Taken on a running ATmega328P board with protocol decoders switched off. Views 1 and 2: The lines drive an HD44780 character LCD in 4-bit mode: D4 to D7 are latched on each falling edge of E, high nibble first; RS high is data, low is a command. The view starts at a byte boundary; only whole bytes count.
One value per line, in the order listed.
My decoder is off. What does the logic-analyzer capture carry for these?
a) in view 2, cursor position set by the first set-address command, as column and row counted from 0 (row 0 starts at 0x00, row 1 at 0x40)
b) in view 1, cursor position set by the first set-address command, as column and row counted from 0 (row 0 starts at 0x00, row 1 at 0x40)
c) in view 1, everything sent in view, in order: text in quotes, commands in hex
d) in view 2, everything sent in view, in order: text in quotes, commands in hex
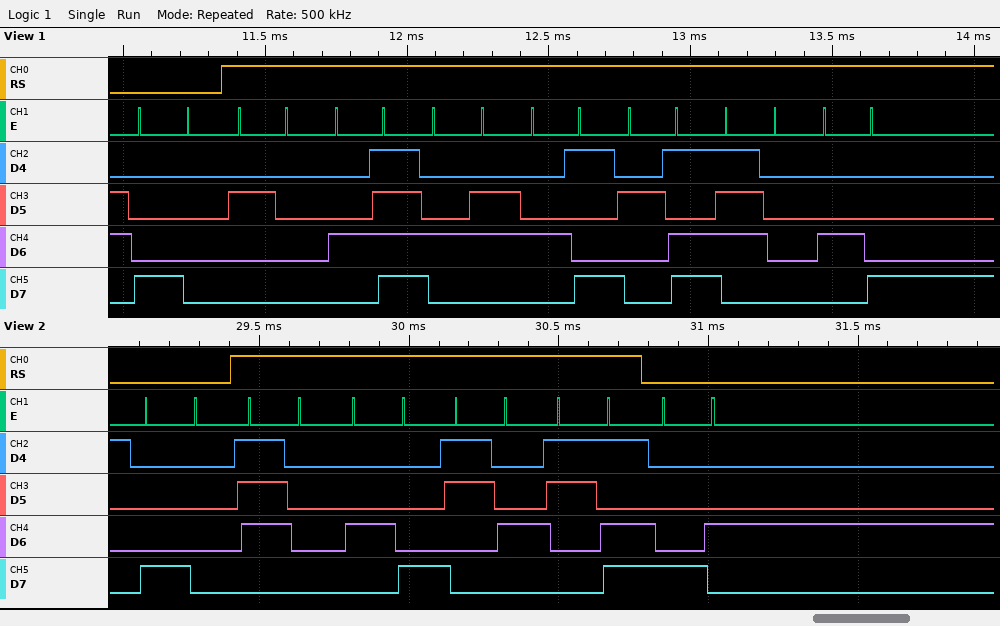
column 0, row 0
column 0, row 0
0x80 " OFI-pH"
0x80 "pH4=" 0x84
